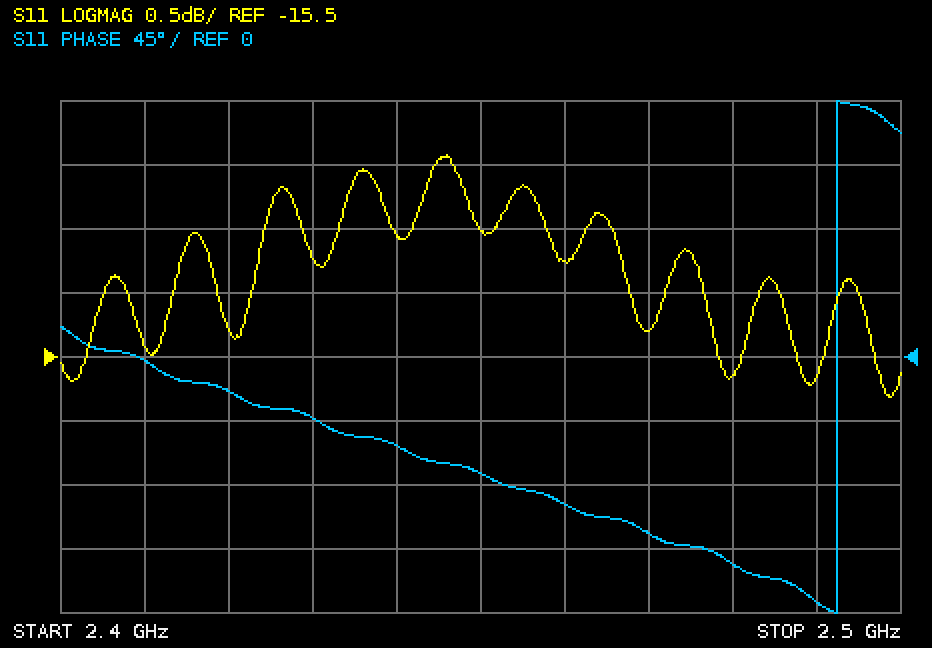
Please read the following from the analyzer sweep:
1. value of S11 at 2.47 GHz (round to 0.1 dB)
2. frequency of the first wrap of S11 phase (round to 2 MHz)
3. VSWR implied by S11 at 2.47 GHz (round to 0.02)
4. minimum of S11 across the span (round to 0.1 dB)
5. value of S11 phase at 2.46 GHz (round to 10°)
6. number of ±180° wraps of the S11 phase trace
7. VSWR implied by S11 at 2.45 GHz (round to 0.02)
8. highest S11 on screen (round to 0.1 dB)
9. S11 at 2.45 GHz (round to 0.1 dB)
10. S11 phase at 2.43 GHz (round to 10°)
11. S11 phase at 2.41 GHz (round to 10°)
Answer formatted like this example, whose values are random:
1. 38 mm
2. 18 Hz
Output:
1. -15.3 dB
2. 2.492 GHz
3. 1.42
4. -15.8 dB
5. -100°
6. 1
7. 1.46
8. -13.9 dB
9. -14.5 dB
10. -40°
11. 0°
